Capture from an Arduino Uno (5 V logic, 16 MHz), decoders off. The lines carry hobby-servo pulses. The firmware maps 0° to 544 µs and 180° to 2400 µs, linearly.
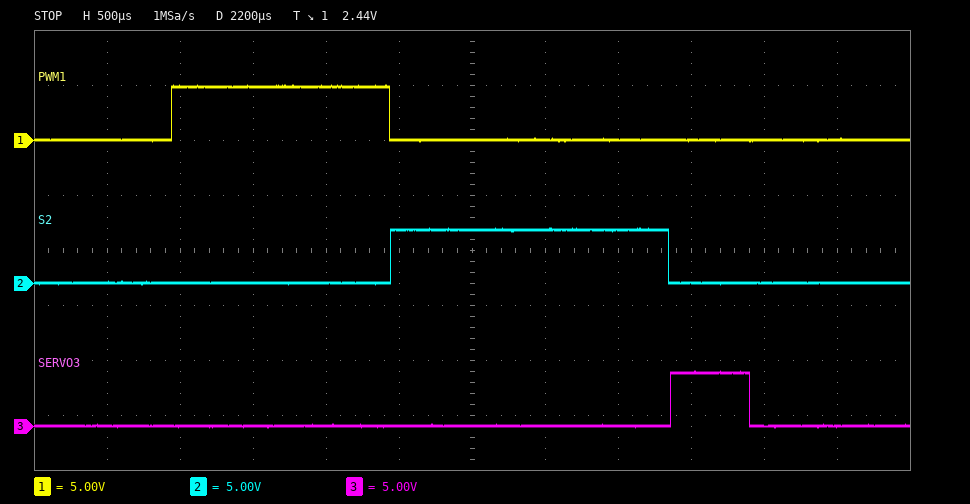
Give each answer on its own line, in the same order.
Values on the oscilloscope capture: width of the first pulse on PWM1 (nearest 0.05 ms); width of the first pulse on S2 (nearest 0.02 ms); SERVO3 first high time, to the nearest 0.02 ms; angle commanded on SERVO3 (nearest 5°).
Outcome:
1.50 ms
1.90 ms
0.54 ms
0°
